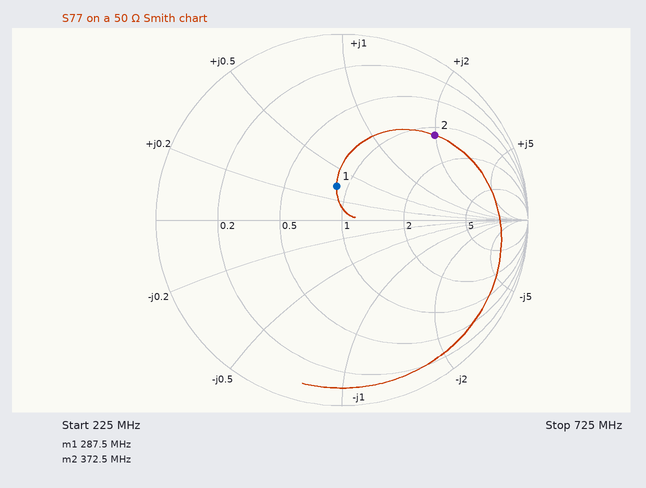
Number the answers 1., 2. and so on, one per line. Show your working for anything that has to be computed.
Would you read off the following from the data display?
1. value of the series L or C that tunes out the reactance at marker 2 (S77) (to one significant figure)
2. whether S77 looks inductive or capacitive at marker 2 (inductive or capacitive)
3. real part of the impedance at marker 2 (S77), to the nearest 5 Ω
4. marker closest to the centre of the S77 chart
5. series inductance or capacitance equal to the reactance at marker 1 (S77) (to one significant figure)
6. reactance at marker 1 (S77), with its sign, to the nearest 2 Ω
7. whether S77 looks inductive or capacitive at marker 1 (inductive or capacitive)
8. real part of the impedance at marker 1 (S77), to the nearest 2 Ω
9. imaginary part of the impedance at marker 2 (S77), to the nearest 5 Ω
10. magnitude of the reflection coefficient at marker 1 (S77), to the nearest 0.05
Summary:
1. C = 1/(2π × 372.5 MHz × 100 Ω) ≈ 4 pF
2. inductive
3. 60 Ω
4. marker 1
5. L = 16 Ω/(2π × 287.5 MHz) ≈ 9 nH
6. +16 Ω
7. inductive
8. 44 Ω
9. +100 Ω
10. 0.20
